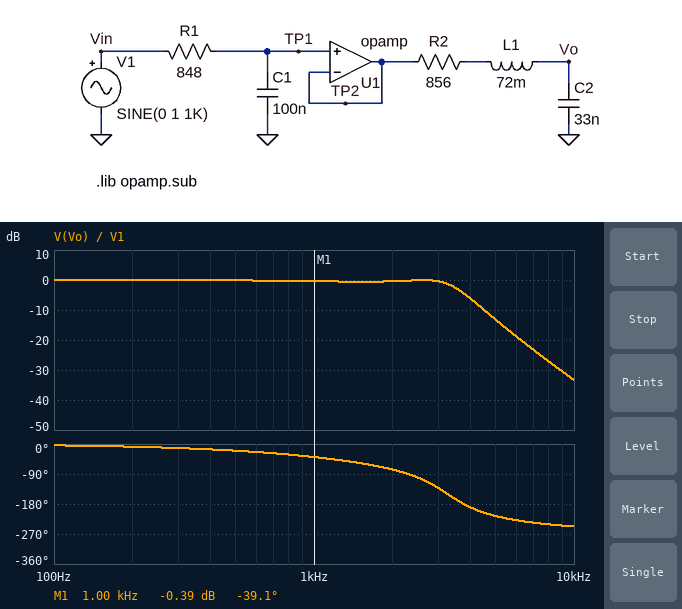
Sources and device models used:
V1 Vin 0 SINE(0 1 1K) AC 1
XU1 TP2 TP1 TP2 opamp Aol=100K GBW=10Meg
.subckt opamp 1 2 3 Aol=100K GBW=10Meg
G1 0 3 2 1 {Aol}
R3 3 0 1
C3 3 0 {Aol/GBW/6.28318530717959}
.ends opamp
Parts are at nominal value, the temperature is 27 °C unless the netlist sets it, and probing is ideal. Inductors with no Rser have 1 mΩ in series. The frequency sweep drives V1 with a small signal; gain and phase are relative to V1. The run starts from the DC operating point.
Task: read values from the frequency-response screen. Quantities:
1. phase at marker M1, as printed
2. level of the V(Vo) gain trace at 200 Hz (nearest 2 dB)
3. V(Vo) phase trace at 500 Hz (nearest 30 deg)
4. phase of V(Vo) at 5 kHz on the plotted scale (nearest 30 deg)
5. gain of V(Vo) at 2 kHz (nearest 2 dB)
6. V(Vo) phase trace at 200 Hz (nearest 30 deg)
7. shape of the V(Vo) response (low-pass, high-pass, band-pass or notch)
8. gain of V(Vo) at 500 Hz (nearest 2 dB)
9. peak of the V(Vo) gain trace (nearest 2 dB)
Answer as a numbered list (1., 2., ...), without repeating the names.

1. -39.1 deg
2. 0 dB
3. -30 deg
4. -210 deg
5. 0 dB
6. 0 deg
7. low-pass
8. 0 dB
9. 0 dB
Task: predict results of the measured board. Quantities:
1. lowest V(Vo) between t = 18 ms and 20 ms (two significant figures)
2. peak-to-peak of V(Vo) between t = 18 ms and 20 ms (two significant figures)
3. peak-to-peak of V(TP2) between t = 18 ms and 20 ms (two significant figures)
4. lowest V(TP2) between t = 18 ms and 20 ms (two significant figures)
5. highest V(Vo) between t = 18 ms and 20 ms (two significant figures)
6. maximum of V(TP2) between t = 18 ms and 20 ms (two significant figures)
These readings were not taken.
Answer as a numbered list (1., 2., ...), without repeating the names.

1. -960 mV
2. 1.9 V
3. 1.8 V
4. -880 mV
5. 960 mV
6. 880 mV
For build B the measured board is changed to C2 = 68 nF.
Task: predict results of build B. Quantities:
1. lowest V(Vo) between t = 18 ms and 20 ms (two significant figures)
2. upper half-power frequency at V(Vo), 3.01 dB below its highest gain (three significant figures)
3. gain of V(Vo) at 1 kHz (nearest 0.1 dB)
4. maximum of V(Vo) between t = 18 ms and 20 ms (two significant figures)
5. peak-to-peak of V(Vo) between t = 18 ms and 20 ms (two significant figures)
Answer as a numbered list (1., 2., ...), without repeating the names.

1. -1.0 V
2. 2.38 kHz
3. 0 dB
4. 1.0 V
5. 2.0 V
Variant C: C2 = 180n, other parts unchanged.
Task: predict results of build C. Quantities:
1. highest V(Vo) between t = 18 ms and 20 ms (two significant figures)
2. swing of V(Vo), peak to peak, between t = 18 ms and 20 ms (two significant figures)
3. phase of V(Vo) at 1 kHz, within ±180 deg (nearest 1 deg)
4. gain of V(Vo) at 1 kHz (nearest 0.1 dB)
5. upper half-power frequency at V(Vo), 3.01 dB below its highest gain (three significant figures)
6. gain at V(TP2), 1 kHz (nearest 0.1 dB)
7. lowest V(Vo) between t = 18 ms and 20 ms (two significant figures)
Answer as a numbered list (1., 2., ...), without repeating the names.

1. 810 mV
2. 1.6 V
3. -91 deg
4. -1.8 dB
5. 1.20 kHz
6. -1.1 dB
7. -810 mV
